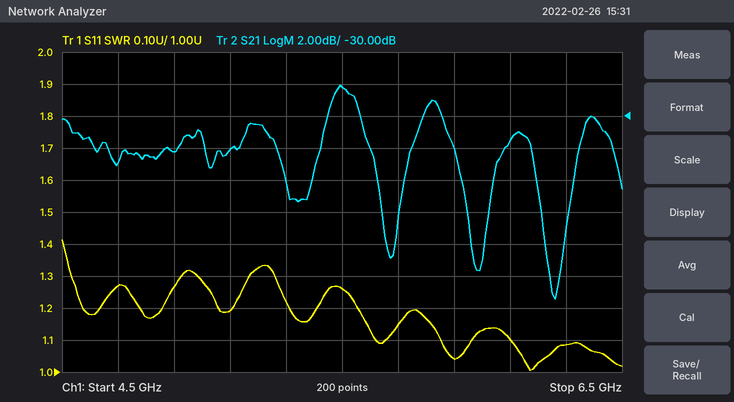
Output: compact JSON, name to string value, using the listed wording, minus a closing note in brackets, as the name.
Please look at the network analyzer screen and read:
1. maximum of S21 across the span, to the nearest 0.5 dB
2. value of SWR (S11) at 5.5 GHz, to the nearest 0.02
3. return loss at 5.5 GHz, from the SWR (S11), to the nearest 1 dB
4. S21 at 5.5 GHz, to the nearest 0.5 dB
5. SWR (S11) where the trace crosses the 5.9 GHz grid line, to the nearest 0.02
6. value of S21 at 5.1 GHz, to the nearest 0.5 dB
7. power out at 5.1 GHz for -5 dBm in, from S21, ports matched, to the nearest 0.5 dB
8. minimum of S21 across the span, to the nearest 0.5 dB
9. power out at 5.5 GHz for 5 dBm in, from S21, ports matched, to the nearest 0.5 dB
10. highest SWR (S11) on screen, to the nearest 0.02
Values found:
{"maximum of S21 across the span, to the nearest 0.5 dB": "-28.0 dB", "value of SWR (S11) at 5.5 GHz, to the nearest 0.02": "1.26", "return loss at 5.5 GHz, from the SWR (S11), to the nearest 1 dB": "19 dB", "S21 at 5.5 GHz, to the nearest 0.5 dB": "-28.0 dB", "SWR (S11) where the trace crosses the 5.9 GHz grid line, to the nearest 0.02": "1.04", "value of S21 at 5.1 GHz, to the nearest 0.5 dB": "-32.0 dB", "power out at 5.1 GHz for -5 dBm in, from S21, ports matched, to the nearest 0.5 dB": "-37.0 dBm", "minimum of S21 across the span, to the nearest 0.5 dB": "-41.5 dB", "power out at 5.5 GHz for 5 dBm in, from S21, ports matched, to the nearest 0.5 dB": "-23.0 dBm", "highest SWR (S11) on screen, to the nearest 0.02": "1.42"}
